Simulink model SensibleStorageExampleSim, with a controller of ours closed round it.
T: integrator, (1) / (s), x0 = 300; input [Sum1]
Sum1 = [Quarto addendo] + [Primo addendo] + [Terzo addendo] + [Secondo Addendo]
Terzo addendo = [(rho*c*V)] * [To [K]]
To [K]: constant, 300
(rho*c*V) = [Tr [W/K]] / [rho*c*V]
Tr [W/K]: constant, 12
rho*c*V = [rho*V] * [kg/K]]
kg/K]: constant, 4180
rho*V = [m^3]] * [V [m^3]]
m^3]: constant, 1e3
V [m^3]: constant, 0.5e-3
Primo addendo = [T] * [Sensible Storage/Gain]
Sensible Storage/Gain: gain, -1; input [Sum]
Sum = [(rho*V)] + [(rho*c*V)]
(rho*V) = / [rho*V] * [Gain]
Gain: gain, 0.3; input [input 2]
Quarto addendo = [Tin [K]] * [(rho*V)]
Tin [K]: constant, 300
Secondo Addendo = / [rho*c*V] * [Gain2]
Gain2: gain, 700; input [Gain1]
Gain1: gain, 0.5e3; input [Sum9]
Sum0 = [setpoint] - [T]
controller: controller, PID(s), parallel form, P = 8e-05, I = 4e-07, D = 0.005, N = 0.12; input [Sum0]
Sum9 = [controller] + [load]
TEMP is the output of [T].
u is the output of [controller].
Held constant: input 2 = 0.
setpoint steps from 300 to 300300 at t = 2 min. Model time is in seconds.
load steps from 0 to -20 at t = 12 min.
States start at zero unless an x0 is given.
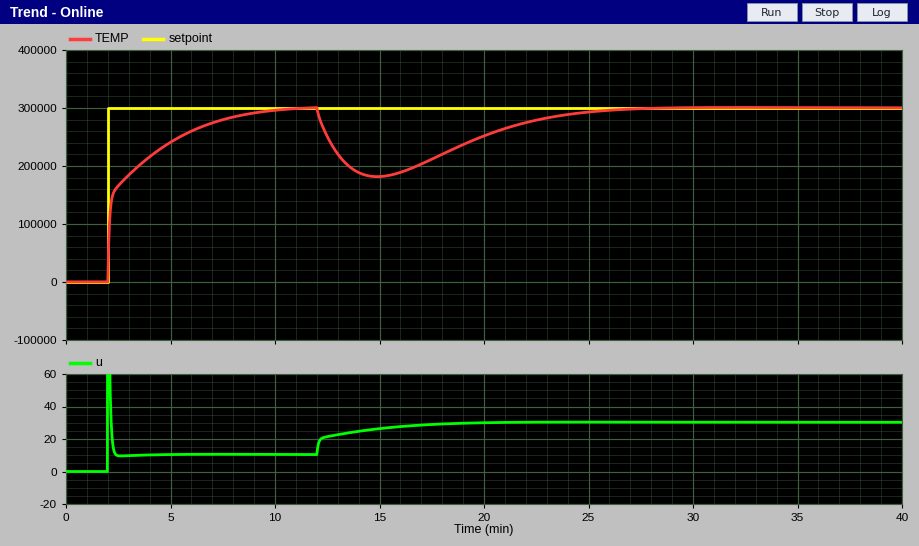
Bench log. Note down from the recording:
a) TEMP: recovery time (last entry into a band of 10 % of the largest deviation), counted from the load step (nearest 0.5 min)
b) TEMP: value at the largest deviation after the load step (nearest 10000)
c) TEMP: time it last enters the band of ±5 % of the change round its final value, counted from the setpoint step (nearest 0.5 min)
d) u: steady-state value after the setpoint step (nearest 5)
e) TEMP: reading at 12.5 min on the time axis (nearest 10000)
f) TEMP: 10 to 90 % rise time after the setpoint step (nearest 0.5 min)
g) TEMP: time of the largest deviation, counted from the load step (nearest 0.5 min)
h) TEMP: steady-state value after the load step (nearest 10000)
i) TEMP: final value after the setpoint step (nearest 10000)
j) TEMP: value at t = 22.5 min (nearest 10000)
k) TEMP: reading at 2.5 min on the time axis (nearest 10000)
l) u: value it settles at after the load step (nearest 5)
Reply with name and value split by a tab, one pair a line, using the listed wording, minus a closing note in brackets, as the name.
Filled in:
TEMP: recovery time (last entry into a band of 10 % of the largest deviation), counted from the load step	12.0 min
TEMP: value at the largest deviation after the load step	180000
TEMP: time it last enters the band of ±5 % of the change round its final value, counted from the setpoint step	6.0 min
u: steady-state value after the setpoint step	10
TEMP: reading at 12.5 min on the time axis	250000
TEMP: 10 to 90 % rise time after the setpoint step	4.5 min
TEMP: time of the largest deviation, counted from the load step	3.0 min
TEMP: steady-state value after the load step	300000
TEMP: final value after the setpoint step	300000
TEMP: value at t = 22.5 min	280000
TEMP: reading at 2.5 min on the time axis	170000
u: value it settles at after the load step	30
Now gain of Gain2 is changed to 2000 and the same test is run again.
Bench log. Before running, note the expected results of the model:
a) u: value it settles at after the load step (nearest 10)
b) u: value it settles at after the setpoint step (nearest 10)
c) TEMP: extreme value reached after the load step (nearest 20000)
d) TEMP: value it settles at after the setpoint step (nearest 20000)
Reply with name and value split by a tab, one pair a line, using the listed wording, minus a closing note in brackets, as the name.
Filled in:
u: value it settles at after the load step	20
u: value it settles at after the setpoint step	0
TEMP: extreme value reached after the load step	160000
TEMP: value it settles at after the setpoint step	300000
